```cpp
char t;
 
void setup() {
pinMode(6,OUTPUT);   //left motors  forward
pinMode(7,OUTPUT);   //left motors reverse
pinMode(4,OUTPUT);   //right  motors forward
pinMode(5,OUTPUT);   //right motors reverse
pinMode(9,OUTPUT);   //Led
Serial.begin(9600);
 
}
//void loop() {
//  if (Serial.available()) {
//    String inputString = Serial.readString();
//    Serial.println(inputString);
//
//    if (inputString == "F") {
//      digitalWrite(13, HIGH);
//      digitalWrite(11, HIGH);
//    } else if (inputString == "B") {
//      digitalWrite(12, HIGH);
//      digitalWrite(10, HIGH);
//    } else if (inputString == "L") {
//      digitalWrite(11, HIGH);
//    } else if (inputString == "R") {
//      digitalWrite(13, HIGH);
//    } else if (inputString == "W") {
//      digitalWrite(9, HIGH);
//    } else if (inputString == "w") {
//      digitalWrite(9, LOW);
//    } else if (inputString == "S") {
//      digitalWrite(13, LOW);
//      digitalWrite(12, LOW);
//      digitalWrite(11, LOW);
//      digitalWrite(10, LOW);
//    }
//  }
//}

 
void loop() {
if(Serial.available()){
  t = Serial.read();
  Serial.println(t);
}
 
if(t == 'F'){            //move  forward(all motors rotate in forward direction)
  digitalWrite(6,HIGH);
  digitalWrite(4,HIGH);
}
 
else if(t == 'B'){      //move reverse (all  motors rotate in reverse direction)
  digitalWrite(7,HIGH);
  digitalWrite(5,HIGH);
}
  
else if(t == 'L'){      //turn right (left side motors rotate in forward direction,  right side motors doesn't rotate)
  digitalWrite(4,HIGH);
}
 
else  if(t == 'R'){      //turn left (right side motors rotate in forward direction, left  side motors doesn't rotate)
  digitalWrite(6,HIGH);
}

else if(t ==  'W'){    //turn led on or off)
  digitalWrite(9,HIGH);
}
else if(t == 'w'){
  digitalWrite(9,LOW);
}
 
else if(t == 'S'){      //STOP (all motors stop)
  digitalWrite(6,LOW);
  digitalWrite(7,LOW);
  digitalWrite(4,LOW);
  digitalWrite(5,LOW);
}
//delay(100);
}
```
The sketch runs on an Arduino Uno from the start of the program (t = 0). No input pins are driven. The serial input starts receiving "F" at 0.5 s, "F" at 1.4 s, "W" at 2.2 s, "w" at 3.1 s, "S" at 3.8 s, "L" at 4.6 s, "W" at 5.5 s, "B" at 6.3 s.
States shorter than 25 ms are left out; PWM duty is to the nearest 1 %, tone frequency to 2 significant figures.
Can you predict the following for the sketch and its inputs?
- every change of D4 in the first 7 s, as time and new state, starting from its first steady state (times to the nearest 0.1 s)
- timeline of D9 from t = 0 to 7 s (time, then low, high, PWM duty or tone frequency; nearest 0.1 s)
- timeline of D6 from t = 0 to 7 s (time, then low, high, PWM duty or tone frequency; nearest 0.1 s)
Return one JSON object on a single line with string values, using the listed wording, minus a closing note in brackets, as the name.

{"every change of D4 in the first 7 s, as time and new state, starting from its first steady state": "0 s low; 0.5 s high; 3.8 s low; 4.6 s high", "timeline of D9 from t = 0 to 7 s": "0 s low; 2.2 s high; 3.1 s low; 5.5 s high", "timeline of D6 from t = 0 to 7 s": "0 s low; 0.5 s high; 3.8 s low"}
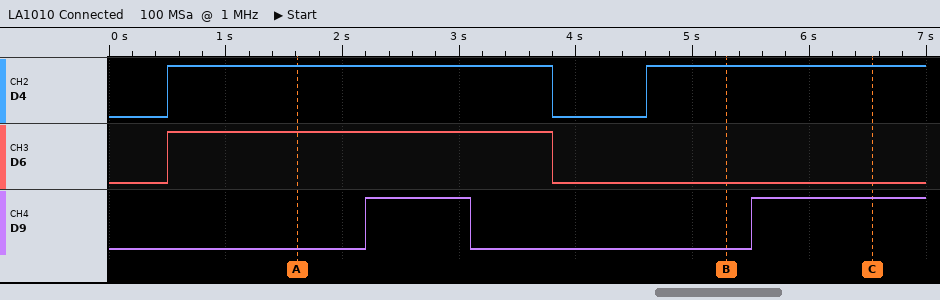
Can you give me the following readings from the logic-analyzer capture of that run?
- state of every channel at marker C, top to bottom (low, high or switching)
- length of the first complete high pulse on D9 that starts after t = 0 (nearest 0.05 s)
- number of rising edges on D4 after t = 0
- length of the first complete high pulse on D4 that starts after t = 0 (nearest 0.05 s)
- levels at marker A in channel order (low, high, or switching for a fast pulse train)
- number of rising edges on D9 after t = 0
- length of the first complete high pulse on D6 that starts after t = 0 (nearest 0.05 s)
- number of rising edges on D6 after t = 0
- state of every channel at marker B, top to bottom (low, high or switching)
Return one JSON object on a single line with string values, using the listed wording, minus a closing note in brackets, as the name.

{"state of every channel at marker C, top to bottom": "D4 high, D6 low, D9 high", "length of the first complete high pulse on D9 that starts after t = 0": "0.90 s", "number of rising edges on D4 after t = 0": "2", "length of the first complete high pulse on D4 that starts after t = 0": "3.30 s", "levels at marker A in channel order": "D4 high, D6 high, D9 low", "number of rising edges on D9 after t = 0": "2", "length of the first complete high pulse on D6 that starts after t = 0": "3.30 s", "number of rising edges on D6 after t = 0": "1", "state of every channel at marker B, top to bottom": "D4 high, D6 low, D9 low"}
